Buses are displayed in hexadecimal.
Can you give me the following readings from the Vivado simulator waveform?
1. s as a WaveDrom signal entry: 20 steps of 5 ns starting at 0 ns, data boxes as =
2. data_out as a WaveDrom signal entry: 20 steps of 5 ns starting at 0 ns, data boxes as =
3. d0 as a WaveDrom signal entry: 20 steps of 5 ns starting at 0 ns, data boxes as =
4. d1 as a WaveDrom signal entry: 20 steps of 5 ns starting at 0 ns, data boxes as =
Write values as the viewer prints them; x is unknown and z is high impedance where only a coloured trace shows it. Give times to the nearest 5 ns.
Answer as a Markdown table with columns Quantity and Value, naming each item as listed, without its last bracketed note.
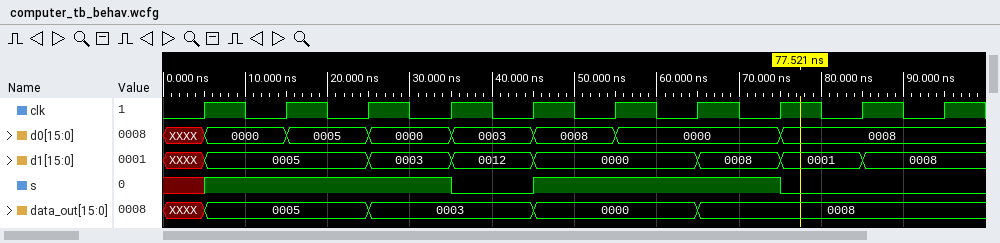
| Quantity | Value |
|---|---|
| s as a WaveDrom signal entry: 20 steps of 5 ns starting at 0 ns, data boxes as = | {name: 's', wave: 'x1.....0.1.....0....'} |
| data_out as a WaveDrom signal entry: 20 steps of 5 ns starting at 0 ns, data boxes as = | {name: 'data_out', wave: 'x=...=...=...=......', data: '0005 0003 0000 0008'} |
| d0 as a WaveDrom signal entry: 20 steps of 5 ns starting at 0 ns, data boxes as = | {name: 'd0', wave: 'x=.=.=.=.=.=...=....', data: '0000 0005 0000 0003 0008 0000 0008'} |
| d1 as a WaveDrom signal entry: 20 steps of 5 ns starting at 0 ns, data boxes as = | {name: 'd1', wave: 'x=...=.=.=...=.=.=..', data: '0005 0003 0012 0000 0008 0001 0008'} |
